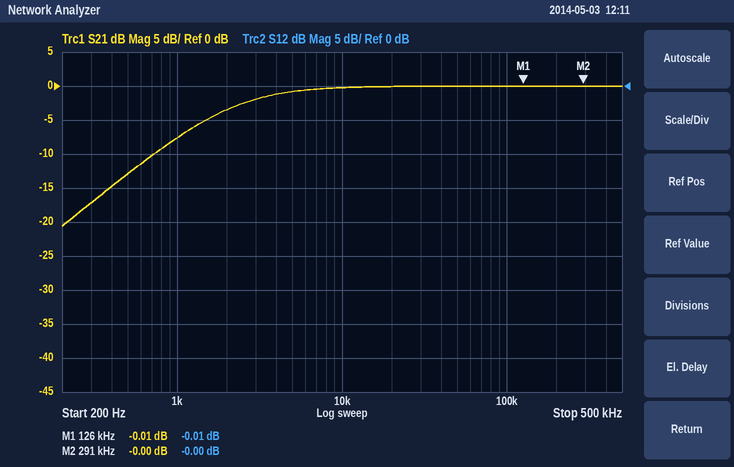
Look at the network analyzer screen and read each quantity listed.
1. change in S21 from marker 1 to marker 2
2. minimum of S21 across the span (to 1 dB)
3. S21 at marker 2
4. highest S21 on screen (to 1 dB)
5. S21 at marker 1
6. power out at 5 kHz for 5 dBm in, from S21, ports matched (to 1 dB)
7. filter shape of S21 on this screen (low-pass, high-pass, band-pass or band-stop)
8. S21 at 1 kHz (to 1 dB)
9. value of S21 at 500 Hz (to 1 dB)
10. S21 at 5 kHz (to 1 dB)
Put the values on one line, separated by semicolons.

0.01 dB; -21 dB; -0.00 dB; 0 dB; -0.01 dB; 4 dBm; high-pass; -8 dB; -13 dB; -1 dB
